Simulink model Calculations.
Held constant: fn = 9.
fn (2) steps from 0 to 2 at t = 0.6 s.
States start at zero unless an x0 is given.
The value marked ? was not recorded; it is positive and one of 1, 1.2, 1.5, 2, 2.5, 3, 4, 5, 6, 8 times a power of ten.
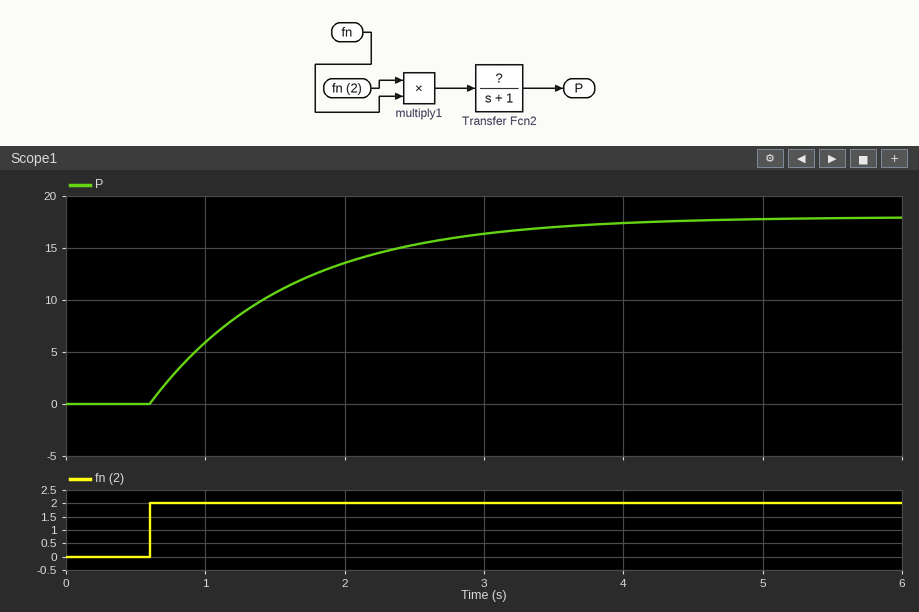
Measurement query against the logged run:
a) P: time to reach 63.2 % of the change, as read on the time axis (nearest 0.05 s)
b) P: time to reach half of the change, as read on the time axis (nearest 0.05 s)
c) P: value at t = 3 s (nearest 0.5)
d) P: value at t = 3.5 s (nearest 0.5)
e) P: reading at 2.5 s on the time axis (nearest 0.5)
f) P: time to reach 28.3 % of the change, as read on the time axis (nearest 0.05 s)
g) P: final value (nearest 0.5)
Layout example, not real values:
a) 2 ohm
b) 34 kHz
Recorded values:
a) 1.60 s
b) 1.30 s
c) 16.5
d) 17.0
e) 15.5
f) 0.95 s
g) 18.0
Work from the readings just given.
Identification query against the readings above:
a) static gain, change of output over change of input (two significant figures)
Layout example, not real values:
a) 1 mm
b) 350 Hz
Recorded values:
a) 9.0
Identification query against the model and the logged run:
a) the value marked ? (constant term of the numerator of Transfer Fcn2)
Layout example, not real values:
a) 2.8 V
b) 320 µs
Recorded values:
a) 1
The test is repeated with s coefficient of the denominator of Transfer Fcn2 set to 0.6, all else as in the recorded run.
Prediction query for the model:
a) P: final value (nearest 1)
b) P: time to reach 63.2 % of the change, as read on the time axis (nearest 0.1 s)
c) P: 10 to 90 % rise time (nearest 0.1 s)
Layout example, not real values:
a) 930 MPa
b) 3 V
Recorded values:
a) 18
b) 1.2 s
c) 1.3 s
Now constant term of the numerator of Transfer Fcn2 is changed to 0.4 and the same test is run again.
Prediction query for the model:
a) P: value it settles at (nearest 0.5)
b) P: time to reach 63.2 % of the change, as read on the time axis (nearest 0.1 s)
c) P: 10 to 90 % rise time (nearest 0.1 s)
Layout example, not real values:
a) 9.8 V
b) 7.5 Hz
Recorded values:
a) 7.0
b) 1.6 s
c) 2.2 s
